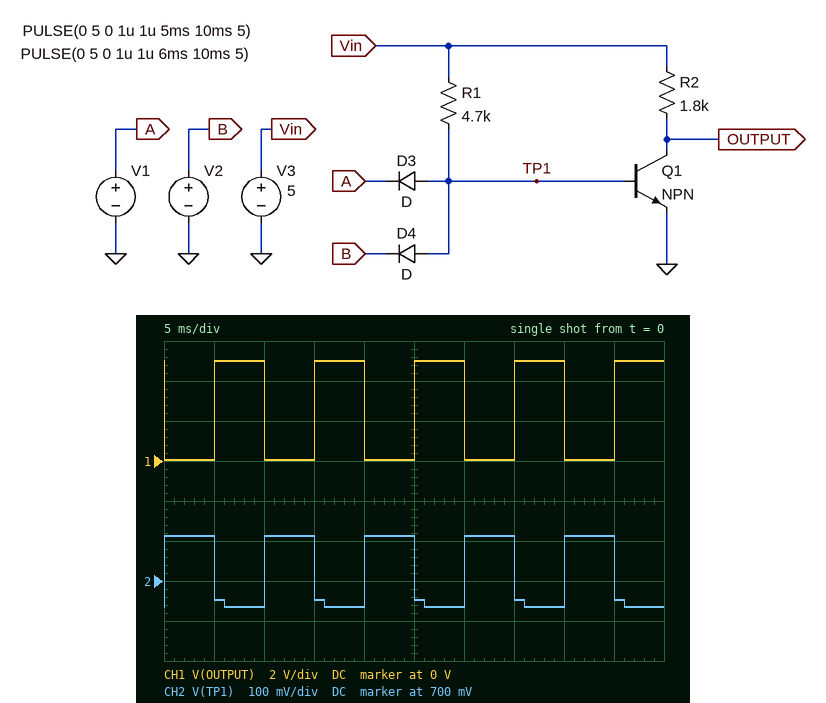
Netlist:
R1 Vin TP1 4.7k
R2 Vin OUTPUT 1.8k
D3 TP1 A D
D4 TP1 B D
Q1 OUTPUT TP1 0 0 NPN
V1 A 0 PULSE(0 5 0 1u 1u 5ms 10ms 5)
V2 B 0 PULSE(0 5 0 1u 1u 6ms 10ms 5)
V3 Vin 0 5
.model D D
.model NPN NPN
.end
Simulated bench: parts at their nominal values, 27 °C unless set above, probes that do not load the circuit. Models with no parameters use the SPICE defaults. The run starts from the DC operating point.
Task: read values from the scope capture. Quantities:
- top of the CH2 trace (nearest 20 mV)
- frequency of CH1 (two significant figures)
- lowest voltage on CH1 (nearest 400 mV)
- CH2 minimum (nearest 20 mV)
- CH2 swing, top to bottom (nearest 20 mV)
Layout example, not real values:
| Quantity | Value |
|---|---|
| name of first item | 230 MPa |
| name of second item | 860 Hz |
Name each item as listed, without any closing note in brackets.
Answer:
| Quantity | Value |
|---|---|
| top of the CH2 trace | 820 mV |
| frequency of CH1 | 100 Hz |
| lowest voltage on CH1 | 0 V |
| CH2 minimum | 640 mV |
| CH2 swing, top to bottom | 180 mV |
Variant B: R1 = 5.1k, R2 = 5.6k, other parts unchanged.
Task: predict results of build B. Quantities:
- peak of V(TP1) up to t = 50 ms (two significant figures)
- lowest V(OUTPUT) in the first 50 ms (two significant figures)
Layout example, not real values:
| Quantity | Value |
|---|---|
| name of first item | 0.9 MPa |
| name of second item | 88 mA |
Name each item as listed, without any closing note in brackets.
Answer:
| Quantity | Value |
|---|---|
| peak of V(TP1) up to t = 50 ms | 800 mV |
| lowest V(OUTPUT) in the first 50 ms | 29 mV |
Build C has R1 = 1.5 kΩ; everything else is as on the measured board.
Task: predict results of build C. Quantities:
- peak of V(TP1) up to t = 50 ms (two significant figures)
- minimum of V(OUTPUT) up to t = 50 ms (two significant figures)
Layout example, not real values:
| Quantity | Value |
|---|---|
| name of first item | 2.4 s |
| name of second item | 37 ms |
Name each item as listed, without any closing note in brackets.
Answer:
| Quantity | Value |
|---|---|
| peak of V(TP1) up to t = 50 ms | 830 mV |
| minimum of V(OUTPUT) up to t = 50 ms | 29 mV |
